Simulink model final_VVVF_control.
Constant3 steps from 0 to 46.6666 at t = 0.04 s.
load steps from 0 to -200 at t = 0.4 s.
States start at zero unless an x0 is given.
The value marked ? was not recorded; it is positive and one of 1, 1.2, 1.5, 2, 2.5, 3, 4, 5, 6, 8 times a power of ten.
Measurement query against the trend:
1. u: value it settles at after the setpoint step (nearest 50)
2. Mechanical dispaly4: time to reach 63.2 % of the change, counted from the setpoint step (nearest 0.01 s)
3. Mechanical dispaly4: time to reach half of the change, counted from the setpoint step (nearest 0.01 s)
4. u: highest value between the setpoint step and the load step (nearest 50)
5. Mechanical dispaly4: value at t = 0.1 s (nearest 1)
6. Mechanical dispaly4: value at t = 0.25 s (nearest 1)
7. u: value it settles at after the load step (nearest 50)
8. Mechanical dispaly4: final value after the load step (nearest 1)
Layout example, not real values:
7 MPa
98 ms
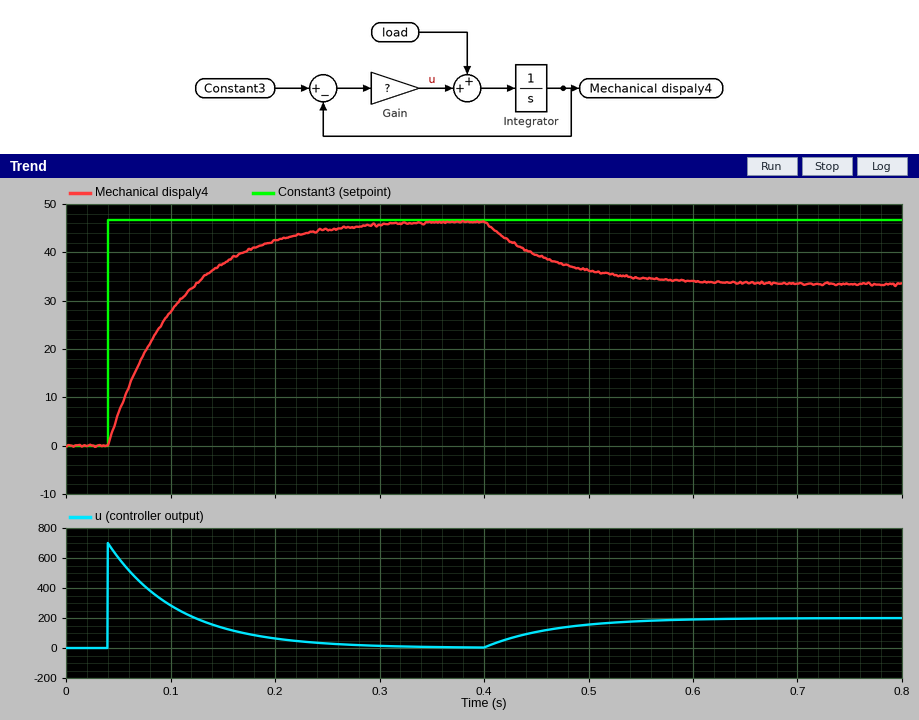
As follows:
0
0.07 s
0.05 s
700
28
45
200
33
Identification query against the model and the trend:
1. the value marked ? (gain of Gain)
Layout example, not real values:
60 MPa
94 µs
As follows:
15
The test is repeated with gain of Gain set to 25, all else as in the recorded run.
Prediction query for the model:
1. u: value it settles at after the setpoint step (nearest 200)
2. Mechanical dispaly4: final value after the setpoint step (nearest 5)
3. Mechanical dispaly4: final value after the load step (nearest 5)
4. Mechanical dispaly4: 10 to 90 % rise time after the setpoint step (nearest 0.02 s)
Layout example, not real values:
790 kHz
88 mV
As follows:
0
45
40
0.08 s
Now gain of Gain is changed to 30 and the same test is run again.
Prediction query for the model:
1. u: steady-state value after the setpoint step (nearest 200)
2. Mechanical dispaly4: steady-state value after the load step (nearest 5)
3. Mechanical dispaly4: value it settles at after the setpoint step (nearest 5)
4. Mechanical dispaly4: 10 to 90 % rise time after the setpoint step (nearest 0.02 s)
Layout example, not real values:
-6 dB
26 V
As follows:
0
40
45
0.08 s
